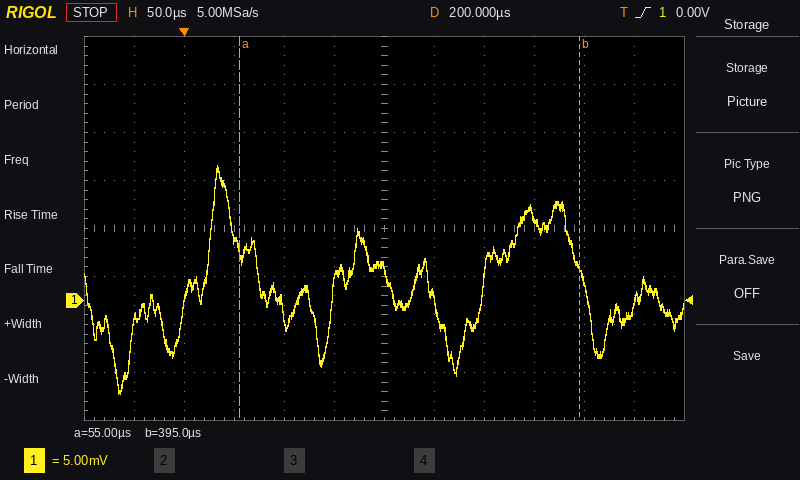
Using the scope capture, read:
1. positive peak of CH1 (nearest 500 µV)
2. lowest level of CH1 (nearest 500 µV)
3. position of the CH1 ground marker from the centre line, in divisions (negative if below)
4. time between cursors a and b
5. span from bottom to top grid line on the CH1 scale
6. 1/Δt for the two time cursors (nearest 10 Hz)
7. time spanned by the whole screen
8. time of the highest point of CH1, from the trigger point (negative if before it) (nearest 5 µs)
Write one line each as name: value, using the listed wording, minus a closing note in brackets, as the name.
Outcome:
positive peak of CH1: 14.0 mV
lowest level of CH1: -9.5 mV
position of the CH1 ground marker from the centre line, in divisions: -1.5 div
time between cursors a and b: 340 µs
span from bottom to top grid line on the CH1 scale: 40 mV
1/Δt for the two time cursors: 2.94 kHz
time spanned by the whole screen: 600 µs
time of the highest point of CH1, from the trigger point (negative if before it): +35 µs
